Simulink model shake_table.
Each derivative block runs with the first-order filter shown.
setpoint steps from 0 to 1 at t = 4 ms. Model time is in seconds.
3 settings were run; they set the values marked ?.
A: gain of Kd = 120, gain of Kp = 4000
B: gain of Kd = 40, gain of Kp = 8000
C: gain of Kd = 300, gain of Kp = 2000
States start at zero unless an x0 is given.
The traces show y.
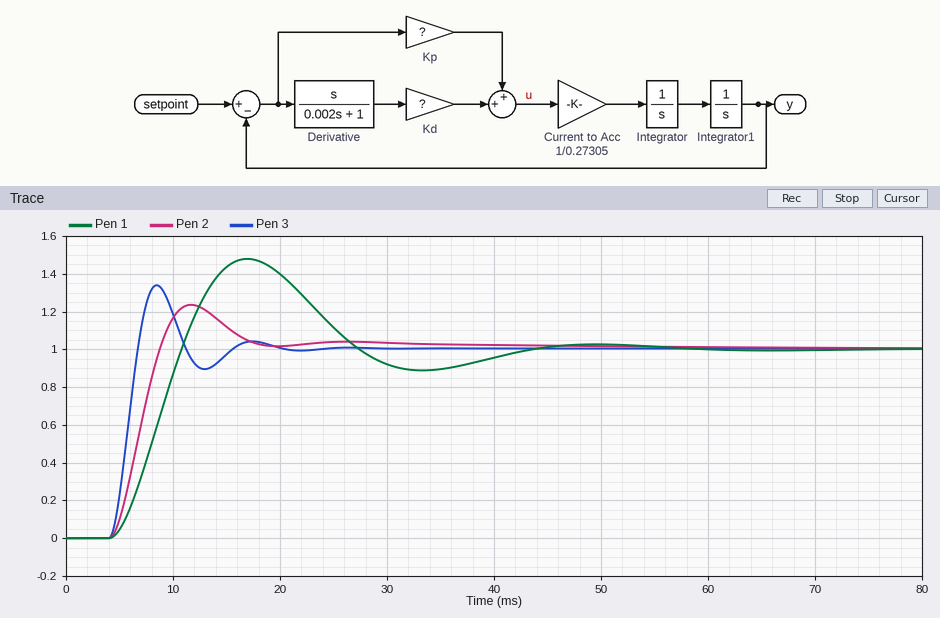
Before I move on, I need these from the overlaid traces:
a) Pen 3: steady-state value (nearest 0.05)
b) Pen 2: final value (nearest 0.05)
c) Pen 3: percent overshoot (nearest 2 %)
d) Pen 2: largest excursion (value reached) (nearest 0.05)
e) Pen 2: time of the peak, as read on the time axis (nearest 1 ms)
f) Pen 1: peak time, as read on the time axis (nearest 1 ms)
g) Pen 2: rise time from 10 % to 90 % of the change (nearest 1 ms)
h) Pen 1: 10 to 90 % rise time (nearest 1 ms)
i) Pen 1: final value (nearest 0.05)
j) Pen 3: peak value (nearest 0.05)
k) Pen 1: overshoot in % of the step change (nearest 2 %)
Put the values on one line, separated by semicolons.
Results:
1.00; 1.00; 34 %; 1.25; 12 ms; 17 ms; 3 ms; 5 ms; 1.00; 1.35; 48 %
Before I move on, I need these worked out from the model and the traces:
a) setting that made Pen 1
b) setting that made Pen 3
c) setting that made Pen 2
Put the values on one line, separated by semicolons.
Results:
B; C; A
